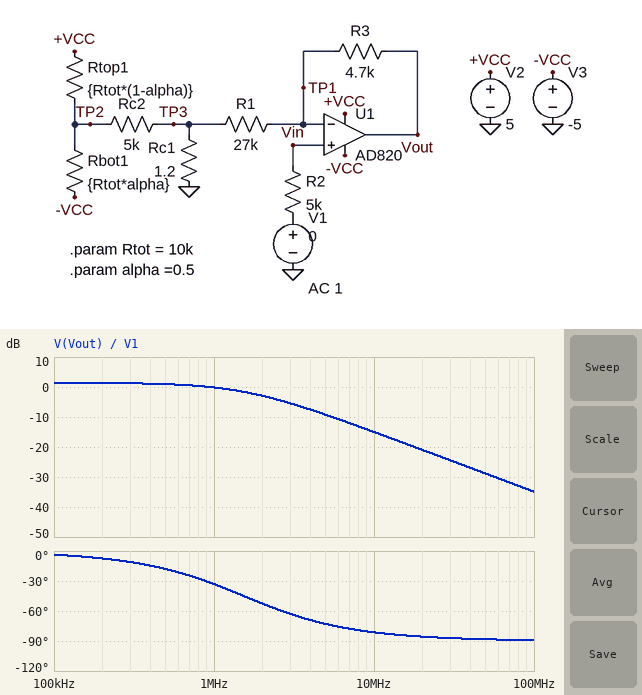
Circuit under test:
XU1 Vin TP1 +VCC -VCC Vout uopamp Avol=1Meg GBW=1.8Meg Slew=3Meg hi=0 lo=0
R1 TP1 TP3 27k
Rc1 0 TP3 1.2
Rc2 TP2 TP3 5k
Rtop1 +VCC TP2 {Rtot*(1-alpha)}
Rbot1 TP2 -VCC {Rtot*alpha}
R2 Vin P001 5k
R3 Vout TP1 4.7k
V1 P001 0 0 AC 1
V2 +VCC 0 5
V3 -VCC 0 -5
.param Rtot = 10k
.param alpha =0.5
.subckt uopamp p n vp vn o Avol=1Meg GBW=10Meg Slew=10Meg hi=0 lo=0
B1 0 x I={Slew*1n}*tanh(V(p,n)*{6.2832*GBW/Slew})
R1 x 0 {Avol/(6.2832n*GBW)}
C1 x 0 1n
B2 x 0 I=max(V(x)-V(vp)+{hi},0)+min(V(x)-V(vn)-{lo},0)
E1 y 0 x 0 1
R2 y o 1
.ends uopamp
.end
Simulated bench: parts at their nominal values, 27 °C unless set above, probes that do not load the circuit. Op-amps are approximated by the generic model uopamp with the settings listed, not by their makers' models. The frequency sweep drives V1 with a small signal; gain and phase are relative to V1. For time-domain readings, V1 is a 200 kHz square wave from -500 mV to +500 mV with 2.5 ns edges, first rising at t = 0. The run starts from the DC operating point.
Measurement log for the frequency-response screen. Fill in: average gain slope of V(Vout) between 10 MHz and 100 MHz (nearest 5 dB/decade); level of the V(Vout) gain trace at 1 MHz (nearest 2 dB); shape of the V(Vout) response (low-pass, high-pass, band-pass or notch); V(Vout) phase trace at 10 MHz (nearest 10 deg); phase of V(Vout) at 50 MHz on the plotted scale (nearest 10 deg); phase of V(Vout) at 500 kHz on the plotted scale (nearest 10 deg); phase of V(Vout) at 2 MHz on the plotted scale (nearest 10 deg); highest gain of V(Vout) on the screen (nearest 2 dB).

-20 dB/decade
0 dB
low-pass
-80 deg
-90 deg
-20 deg
-50 deg
2 dB
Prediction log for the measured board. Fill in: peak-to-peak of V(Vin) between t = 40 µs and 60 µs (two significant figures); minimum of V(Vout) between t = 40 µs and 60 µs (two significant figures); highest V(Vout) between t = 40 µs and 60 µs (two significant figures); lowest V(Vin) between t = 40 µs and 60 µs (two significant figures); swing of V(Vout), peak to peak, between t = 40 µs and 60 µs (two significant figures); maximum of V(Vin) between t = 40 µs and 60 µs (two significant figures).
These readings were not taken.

1.0 V
-590 mV
590 mV
-500 mV
1.2 V
500 mV
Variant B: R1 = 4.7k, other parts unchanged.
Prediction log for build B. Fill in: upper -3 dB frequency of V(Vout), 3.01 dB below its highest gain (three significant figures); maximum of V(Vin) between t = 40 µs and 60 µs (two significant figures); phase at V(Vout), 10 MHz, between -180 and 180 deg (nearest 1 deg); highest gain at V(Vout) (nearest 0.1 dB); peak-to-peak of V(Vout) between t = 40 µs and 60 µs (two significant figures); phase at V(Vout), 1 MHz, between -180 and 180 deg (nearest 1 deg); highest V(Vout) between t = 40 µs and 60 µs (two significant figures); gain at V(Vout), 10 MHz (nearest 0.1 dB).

900 kHz
500 mV
-85 deg
6.0 dB
2.0 V
-48 deg
1.0 V
-14.9 dB
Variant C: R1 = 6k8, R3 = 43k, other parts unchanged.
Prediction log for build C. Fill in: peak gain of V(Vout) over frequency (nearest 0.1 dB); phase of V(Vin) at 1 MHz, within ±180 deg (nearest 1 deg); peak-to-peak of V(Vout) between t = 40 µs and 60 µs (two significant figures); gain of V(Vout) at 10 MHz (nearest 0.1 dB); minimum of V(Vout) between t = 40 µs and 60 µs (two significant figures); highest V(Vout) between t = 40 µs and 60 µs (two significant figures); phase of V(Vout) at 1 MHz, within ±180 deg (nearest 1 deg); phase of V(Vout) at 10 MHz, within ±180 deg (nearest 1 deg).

17.3 dB
0 deg
6.1 V
-14.9 dB
-3.0 V
3.0 V
-76 deg
-89 deg
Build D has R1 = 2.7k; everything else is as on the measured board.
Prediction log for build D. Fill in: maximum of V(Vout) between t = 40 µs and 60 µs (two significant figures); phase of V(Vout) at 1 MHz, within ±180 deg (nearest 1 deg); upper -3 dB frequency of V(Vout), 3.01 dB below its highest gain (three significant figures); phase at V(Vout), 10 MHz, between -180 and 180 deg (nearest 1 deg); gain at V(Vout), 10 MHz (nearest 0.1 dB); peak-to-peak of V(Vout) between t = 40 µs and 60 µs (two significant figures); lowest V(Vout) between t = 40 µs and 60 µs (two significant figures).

1.4 V
-57 deg
657 kHz
-86 deg
-14.9 dB
2.7 V
-1.4 V
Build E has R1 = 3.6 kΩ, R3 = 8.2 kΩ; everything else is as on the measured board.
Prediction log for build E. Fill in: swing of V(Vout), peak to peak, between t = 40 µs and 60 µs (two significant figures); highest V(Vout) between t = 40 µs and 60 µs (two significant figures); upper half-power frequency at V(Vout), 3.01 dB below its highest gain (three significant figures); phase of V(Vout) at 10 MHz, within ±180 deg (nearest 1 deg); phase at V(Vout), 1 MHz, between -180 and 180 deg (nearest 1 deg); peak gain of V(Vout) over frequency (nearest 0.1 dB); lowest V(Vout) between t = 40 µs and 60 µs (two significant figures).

3.3 V
1.6 V
549 kHz
-87 deg
-61 deg
10.3 dB
-1.6 V
